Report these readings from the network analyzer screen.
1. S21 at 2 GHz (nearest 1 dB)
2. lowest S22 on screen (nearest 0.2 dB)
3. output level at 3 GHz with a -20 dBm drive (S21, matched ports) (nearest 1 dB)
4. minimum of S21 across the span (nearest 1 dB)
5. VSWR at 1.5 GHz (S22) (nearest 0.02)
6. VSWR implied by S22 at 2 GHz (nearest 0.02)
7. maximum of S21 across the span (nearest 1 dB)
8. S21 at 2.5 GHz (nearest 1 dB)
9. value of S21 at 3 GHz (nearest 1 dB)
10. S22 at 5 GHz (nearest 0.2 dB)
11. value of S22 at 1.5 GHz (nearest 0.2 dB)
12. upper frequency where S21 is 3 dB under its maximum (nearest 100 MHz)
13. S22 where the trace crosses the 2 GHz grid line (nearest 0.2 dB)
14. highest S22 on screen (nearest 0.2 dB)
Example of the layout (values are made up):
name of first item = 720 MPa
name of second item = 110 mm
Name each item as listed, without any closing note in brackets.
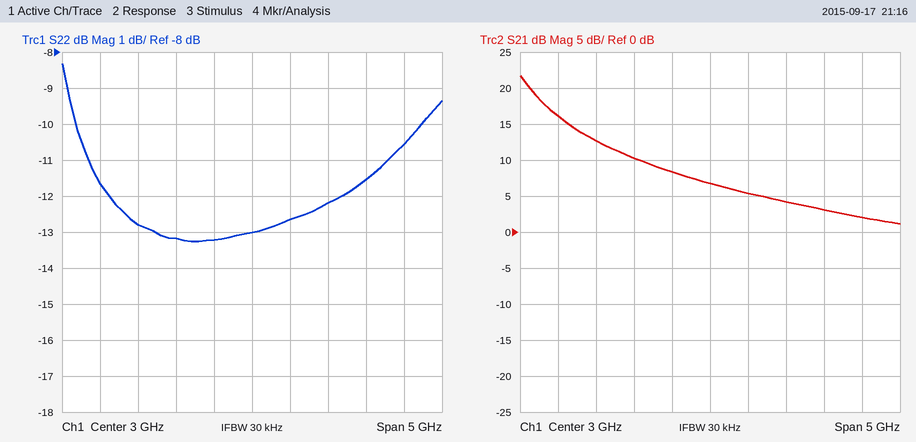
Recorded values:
S21 at 2 GHz = 10 dB
lowest S22 on screen = -13.2 dB
output level at 3 GHz with a -20 dBm drive (S21, matched ports) = -13 dBm
minimum of S21 across the span = 1 dB
VSWR at 1.5 GHz (S22) = 1.60
VSWR implied by S22 at 2 GHz = 1.56
maximum of S21 across the span = 22 dB
S21 at 2.5 GHz = 8 dB
value of S21 at 3 GHz = 7 dB
S22 at 5 GHz = -10.6 dB
value of S22 at 1.5 GHz = -12.8 dB
upper frequency where S21 is 3 dB under its maximum = 700 MHz
S22 where the trace crosses the 2 GHz grid line = -13.2 dB
highest S22 on screen = -8.4 dB
